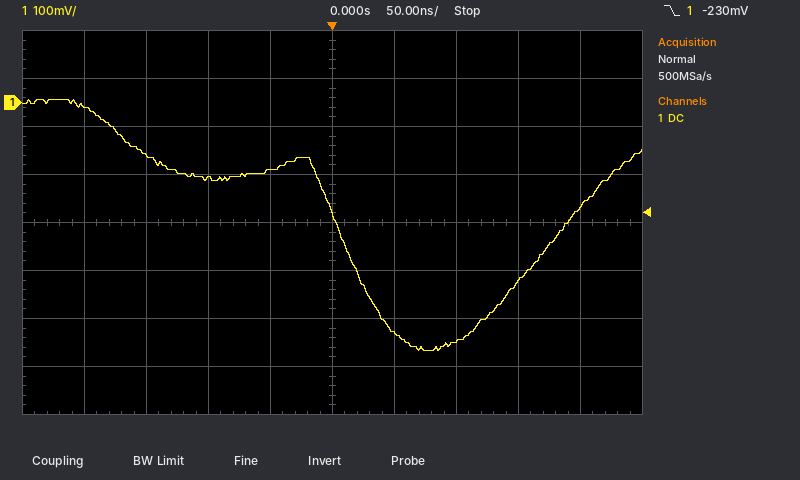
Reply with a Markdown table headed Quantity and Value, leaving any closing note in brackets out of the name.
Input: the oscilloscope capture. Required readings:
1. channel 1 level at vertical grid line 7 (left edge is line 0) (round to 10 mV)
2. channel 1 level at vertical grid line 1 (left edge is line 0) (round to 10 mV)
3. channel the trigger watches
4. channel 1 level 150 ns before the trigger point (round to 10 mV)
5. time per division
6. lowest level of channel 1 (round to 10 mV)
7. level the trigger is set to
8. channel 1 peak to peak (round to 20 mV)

| Quantity | Value |
|---|---|
| channel 1 level at vertical grid line 7 (left edge is line 0) | -500 mV |
| channel 1 level at vertical grid line 1 (left edge is line 0) | -10 mV |
| channel the trigger watches | channel 1 |
| channel 1 level 150 ns before the trigger point | -110 mV |
| time per division | 50 ns |
| lowest level of channel 1 | -520 mV |
| level the trigger is set to | -230 mV |
| channel 1 peak to peak | 520 mV |
